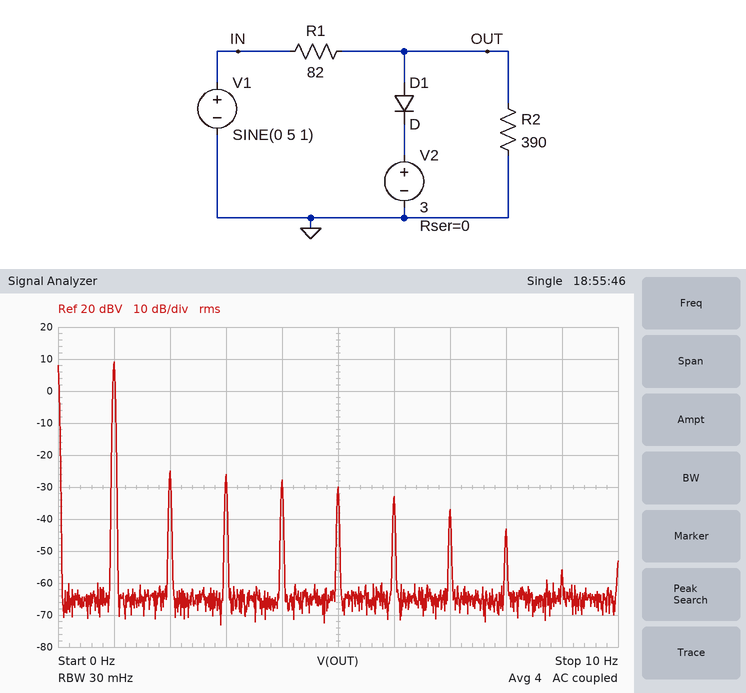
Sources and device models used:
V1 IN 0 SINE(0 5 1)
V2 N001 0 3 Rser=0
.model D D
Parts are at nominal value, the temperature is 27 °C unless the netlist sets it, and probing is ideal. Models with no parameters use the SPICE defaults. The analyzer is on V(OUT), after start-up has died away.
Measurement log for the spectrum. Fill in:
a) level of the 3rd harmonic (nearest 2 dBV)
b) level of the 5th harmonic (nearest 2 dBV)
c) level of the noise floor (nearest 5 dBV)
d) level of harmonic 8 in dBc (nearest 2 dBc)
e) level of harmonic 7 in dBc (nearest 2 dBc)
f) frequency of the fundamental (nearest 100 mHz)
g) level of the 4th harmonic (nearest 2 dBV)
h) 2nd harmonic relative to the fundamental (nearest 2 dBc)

-26 dBV
-30 dBV
-65 dBV
-52 dBc
-46 dBc
1.0 Hz
-28 dBV
-34 dBc
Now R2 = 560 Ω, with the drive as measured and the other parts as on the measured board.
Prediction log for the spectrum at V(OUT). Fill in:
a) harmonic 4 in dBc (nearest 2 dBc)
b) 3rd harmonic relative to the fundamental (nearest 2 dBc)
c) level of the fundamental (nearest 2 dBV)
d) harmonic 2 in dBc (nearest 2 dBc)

-34 dBc
-32 dBc
10 dBV
-30 dBc
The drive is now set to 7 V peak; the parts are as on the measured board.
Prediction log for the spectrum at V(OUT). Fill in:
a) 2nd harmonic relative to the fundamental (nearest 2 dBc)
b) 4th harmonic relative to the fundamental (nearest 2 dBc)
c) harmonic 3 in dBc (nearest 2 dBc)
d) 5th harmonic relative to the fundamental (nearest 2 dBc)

-20 dBc
-30 dBc
-24 dBc
-48 dBc
